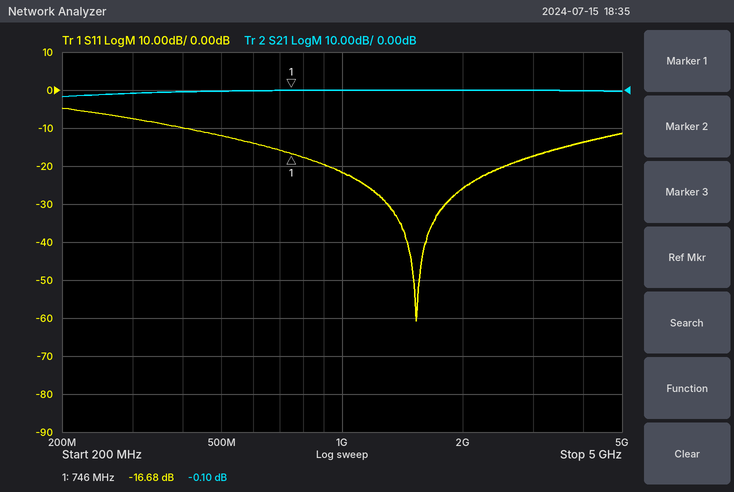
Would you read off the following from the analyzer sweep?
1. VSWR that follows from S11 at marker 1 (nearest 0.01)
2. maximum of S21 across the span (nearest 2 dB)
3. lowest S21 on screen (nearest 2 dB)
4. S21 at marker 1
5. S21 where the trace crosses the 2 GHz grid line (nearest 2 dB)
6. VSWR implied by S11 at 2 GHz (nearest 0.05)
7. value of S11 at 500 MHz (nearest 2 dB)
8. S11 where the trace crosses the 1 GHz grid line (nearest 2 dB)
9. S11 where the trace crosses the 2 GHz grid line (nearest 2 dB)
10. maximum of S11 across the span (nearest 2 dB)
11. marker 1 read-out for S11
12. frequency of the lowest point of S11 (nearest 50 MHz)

1.34
0 dB
-2 dB
-0.10 dB
0 dB
1.10
-12 dB
-22 dB
-26 dB
-4 dB
-16.68 dB
1.55 GHz
